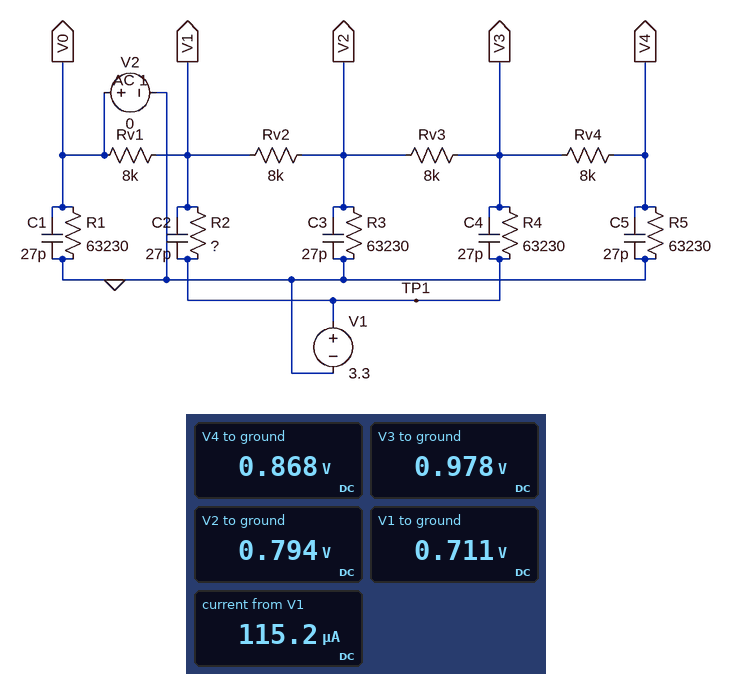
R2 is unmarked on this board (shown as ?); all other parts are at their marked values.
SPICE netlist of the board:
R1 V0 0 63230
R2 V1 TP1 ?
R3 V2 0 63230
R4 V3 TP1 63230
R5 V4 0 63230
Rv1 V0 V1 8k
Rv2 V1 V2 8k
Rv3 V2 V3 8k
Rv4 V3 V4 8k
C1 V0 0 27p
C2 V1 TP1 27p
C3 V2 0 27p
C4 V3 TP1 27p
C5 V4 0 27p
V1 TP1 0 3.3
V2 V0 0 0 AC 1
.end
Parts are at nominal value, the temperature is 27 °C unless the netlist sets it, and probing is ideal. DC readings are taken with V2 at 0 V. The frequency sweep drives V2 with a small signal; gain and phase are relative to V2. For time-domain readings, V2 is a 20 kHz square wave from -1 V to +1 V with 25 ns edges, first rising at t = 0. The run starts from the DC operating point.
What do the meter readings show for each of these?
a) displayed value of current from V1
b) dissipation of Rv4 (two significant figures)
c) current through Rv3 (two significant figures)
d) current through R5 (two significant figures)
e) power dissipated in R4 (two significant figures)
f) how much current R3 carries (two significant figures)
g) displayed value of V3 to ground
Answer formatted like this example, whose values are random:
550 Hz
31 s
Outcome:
115.2 µA
1.5 µW
23 µA
14 µA
85 µW
13 µA
0.978 V
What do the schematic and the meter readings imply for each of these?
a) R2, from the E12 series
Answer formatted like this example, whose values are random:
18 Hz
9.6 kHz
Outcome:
33 kΩ
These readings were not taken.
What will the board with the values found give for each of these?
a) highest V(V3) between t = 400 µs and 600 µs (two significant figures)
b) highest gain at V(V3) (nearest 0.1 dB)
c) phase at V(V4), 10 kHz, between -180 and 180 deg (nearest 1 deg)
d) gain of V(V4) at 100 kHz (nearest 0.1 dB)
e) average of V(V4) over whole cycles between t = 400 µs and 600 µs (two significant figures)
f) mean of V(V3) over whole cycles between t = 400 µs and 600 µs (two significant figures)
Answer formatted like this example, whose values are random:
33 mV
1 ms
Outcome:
1.4 V
-7.7 dB
-4 deg
-9.9 dB
870 mV
980 mV
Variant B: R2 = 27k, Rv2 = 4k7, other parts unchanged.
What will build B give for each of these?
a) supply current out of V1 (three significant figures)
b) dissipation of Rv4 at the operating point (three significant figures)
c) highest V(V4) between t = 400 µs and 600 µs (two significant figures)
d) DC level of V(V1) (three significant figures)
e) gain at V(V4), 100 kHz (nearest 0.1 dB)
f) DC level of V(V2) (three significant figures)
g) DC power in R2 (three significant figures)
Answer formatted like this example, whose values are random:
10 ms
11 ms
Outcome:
128 µA
1.64 µW
1.3 V
806 mV
-9.3 dB
845 mV
230 µW
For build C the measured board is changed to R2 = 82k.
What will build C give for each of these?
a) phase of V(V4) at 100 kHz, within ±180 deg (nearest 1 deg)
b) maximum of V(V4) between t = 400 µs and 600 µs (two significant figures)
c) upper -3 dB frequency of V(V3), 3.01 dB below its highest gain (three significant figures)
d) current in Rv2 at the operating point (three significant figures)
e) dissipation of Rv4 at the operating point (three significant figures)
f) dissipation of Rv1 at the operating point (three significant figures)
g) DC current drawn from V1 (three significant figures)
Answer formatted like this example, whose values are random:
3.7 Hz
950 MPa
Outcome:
-41 deg
1.1 V
178 kHz
18.9 µA
1.03 µW
23.2 µW
74.4 µA
